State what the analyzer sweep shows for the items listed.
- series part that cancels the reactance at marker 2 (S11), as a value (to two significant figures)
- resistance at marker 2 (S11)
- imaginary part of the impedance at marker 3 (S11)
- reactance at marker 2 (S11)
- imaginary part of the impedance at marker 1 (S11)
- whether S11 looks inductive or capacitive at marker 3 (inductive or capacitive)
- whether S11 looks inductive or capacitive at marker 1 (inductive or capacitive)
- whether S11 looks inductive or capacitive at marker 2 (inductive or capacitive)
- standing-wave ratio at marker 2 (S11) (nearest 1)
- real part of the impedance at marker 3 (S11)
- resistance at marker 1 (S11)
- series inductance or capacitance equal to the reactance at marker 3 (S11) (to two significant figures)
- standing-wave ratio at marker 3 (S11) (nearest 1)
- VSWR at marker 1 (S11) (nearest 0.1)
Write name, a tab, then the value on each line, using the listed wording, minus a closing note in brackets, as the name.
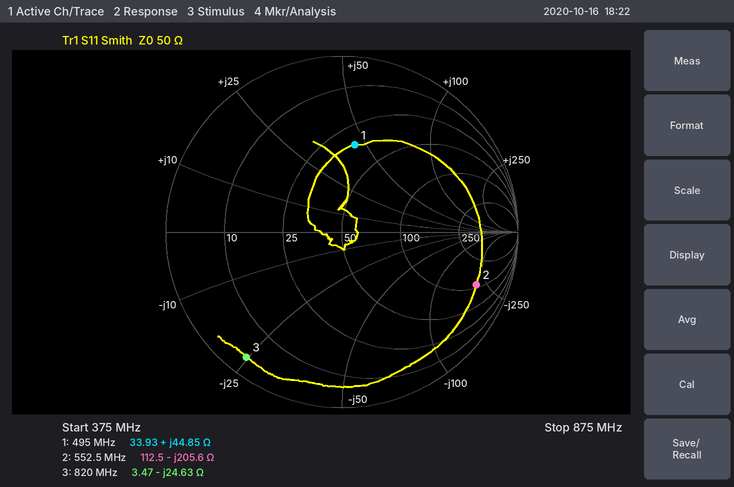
series part that cancels the reactance at marker 2 (S11), as a value	59 nH
resistance at marker 2	112.5 Ω
imaginary part of the impedance at marker 3	-24.63 Ω
reactance at marker 2	-205.6 Ω
imaginary part of the impedance at marker 1	+44.85 Ω
whether S11 looks inductive or capacitive at marker 3	capacitive
whether S11 looks inductive or capacitive at marker 1	inductive
whether S11 looks inductive or capacitive at marker 2	capacitive
standing-wave ratio at marker 2 (S11)	10
real part of the impedance at marker 3	3.47 Ω
resistance at marker 1	33.93 Ω
series inductance or capacitance equal to the reactance at marker 3 (S11)	7.9 pF
standing-wave ratio at marker 3 (S11)	18
VSWR at marker 1 (S11)	3.0
